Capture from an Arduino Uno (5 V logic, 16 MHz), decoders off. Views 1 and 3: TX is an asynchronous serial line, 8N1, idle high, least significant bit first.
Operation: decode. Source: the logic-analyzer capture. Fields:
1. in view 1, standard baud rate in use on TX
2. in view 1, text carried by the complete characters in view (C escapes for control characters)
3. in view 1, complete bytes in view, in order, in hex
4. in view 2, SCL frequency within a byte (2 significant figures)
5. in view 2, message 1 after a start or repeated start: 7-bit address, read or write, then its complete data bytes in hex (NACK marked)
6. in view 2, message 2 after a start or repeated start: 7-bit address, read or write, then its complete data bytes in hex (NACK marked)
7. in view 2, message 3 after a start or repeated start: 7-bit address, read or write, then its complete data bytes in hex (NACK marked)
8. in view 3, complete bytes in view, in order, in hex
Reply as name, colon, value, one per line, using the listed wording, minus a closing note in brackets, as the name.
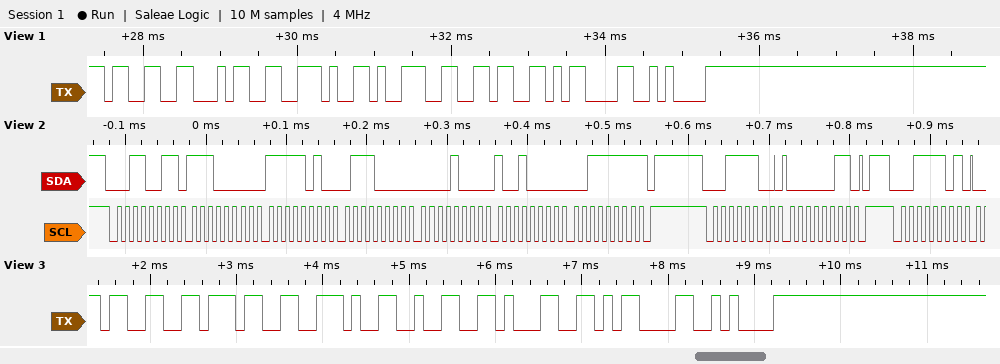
in view 1, standard baud rate in use on TX: 9600 baud
in view 1, text carried by the complete characters in view: "34.96\r\n"
in view 1, complete bytes in view, in order, in hex: 0x33 0x34 0x2E 0x39 0x36 0x0D 0x0A
in view 2, SCL frequency within a byte: 100 kHz
in view 2, message 1 after a start or repeated start: 7-bit address, read or write, then its complete data bytes in hex: 0x19 read: E0 FA 70 08 90 3F NACK
in view 2, message 2 after a start or repeated start: 7-bit address, read or write, then its complete data bytes in hex: 0x1E write: 03
in view 2, message 3 after a start or repeated start: 7-bit address, read or write, then its complete data bytes in hex: 0x1E read
in view 3, complete bytes in view, in order, in hex: 33 37 2E 32 31 0D 0A
